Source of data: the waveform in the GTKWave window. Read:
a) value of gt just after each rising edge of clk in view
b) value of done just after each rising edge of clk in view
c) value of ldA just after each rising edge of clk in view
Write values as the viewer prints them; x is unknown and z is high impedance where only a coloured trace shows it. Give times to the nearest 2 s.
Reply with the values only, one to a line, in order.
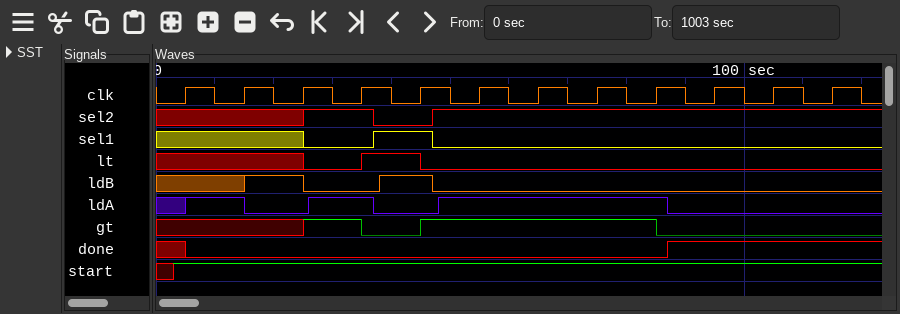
x x 1 0 1 1 1 1 0 0 0 0
0 0 0 0 0 0 0 0 0 1 1 1
1 0 0 1 0 1 1 1 1 0 0 0
